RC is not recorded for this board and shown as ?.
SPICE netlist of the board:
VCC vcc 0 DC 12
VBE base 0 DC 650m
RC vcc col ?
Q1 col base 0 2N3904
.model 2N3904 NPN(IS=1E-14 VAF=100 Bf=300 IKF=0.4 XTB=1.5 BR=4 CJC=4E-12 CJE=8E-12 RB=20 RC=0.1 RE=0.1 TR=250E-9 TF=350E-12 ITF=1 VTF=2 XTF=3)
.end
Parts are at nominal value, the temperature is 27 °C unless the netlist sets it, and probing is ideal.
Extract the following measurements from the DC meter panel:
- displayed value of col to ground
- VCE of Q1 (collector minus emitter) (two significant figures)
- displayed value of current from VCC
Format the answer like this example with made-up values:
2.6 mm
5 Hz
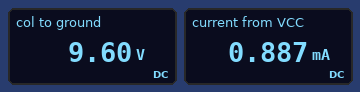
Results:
9.60 V
9.6 V
0.887 mA
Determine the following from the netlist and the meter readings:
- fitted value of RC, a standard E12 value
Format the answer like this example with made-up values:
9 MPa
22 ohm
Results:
2.7 kΩ
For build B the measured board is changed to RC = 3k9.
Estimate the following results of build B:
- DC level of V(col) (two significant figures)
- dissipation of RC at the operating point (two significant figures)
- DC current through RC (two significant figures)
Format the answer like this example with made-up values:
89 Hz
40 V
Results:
8.6 V
3.0 mW
880 µA
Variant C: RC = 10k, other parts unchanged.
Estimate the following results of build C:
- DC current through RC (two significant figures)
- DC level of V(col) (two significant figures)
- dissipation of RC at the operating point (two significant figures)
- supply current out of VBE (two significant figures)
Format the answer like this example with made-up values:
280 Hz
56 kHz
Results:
840 µA
3.6 V
7.0 mW
2.7 µA
